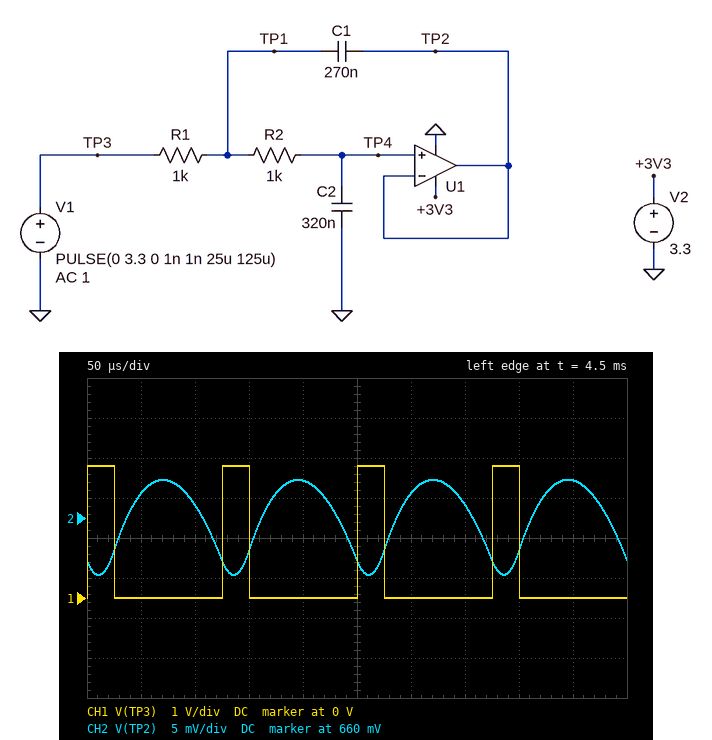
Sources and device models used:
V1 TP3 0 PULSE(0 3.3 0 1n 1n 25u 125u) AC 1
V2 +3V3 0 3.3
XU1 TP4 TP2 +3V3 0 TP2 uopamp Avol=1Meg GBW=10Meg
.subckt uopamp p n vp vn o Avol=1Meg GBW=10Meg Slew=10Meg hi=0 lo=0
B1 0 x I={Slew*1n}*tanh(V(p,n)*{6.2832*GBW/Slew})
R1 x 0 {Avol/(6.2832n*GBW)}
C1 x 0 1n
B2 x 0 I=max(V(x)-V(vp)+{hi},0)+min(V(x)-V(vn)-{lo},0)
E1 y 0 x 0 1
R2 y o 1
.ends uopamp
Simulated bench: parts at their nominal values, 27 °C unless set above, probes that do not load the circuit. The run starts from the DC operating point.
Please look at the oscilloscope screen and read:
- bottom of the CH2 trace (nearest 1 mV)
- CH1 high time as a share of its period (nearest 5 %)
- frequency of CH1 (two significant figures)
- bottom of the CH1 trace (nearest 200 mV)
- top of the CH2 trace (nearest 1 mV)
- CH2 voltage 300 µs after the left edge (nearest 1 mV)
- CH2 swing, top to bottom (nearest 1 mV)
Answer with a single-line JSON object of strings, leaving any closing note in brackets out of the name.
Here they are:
{"bottom of the CH2 trace": "653 mV", "CH1 high time as a share of its period": "20 %", "frequency of CH1": "8.0 kHz", "bottom of the CH1 trace": "0 V", "top of the CH2 trace": "665 mV", "CH2 voltage 300 µs after the left edge": "663 mV", "CH2 swing, top to bottom": "12 mV"}
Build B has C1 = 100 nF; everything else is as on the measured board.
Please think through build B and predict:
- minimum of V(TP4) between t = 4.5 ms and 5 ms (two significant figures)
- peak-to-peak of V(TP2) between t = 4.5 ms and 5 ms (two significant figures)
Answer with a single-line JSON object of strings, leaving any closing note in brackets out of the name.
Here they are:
{"minimum of V(TP4) between t = 4.5 ms and 5 ms": "640 mV", "peak-to-peak of V(TP2) between t = 4.5 ms and 5 ms": "31 mV"}
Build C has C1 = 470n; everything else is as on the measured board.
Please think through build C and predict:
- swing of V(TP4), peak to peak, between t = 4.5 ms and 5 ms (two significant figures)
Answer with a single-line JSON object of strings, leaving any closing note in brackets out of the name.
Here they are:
{"swing of V(TP4), peak to peak, between t = 4.5 ms and 5 ms": "6.9 mV"}
